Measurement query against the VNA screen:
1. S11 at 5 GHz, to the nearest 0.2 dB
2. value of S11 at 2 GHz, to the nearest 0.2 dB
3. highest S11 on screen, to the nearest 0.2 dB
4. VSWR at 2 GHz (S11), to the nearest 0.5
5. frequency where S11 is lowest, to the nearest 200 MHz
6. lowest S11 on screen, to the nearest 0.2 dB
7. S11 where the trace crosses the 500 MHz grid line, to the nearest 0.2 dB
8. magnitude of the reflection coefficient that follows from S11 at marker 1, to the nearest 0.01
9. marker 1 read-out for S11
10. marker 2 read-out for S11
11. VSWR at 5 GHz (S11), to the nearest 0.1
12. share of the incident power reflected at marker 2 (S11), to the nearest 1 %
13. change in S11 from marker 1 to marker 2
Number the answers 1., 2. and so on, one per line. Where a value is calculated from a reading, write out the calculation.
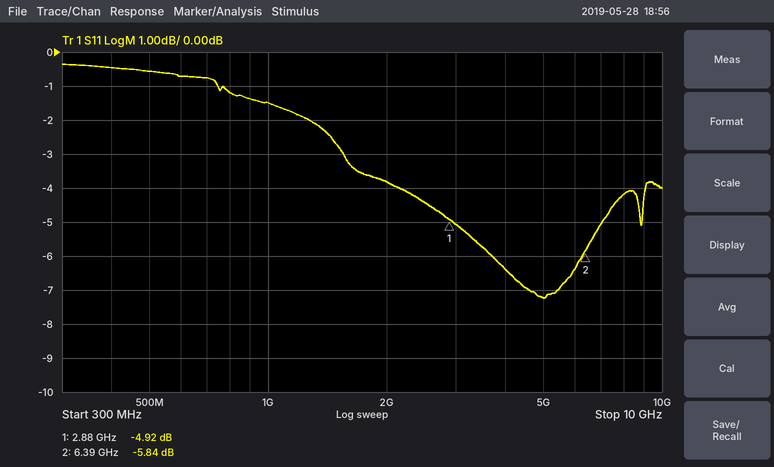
1. -7.2 dB
2. -3.8 dB
3. -0.4 dB
4. |Γ| = 10^(-3.8/20) = 0.6457; VSWR = (1 + 0.6457)/(1 − 0.6457) ≈ 4.64, so 4.5 to the nearest 0.5
5. 5.0 GHz
6. -7.2 dB
7. -0.6 dB
8. 10^(-4.92/20) ≈ 0.57
9. -4.92 dB
10. -5.84 dB
11. |Γ| = 10^(-7.2/20) = 0.4365; VSWR = (1 + 0.4365)/(1 − 0.4365) ≈ 2.5
12. 10^(-5.84/10) ≈ 26 %
13. -5.84 − (-4.92) = -0.92 dB
